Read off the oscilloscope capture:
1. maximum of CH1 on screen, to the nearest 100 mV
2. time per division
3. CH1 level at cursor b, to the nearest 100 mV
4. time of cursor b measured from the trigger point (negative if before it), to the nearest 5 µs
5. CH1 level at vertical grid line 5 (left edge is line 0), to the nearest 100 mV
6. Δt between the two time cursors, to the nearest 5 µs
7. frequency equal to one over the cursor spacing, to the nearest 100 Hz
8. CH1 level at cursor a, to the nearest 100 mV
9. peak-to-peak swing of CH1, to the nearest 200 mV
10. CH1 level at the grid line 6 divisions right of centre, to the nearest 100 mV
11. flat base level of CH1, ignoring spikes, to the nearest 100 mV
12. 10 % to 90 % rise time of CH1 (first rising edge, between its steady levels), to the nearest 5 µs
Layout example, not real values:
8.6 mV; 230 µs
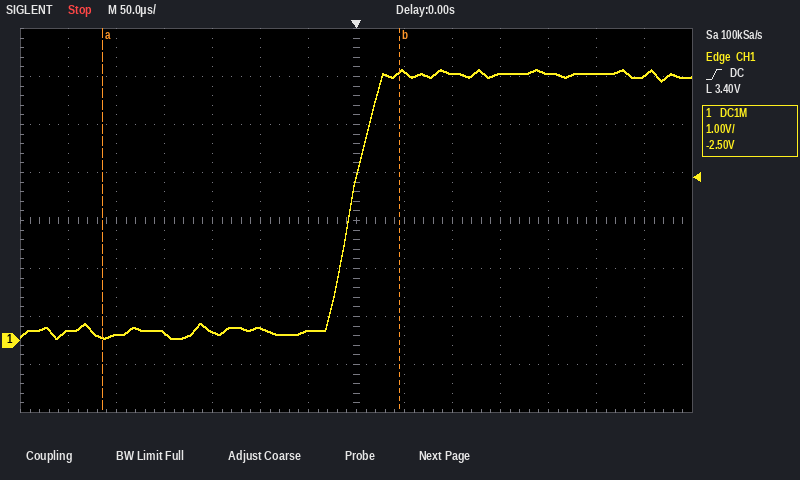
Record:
5.6 V; 50 µs; 5.6 V; +45 µs; 300 mV; 310 µs; 3.2 kHz; 100 mV; 5.6 V; 5.5 V; 200 mV; 45 µs
